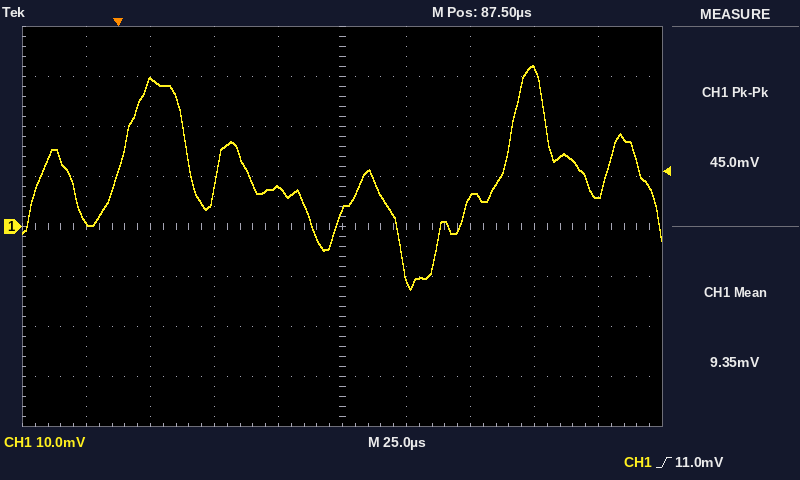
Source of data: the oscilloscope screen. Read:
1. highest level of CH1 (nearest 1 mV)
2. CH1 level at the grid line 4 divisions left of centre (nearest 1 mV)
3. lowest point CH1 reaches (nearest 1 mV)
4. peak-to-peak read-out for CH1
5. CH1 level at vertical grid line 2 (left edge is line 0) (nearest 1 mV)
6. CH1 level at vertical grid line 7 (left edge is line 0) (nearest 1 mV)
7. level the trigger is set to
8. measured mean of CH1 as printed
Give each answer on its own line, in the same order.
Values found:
32 mV
1 mV
-13 mV
45.0 mV
29 mV
6 mV
11.0 mV
9.35 mV
